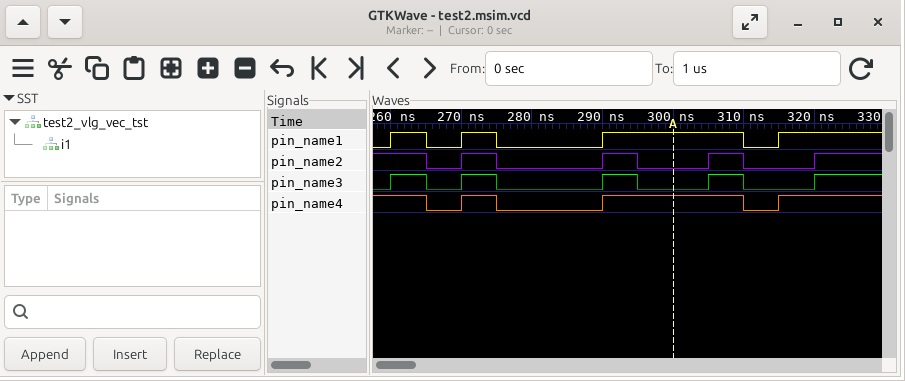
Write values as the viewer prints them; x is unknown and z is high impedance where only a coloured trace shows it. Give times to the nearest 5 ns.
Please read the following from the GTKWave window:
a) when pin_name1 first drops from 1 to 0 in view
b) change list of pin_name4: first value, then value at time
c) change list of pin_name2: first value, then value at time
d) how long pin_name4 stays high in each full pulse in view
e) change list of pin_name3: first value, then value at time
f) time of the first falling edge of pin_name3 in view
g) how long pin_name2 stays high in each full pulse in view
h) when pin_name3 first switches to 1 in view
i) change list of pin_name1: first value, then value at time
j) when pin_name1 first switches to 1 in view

265 ns
1, 0 at 265 ns, 1 at 270 ns, 0 at 275 ns, 1 at 290 ns, 0 at 310 ns, 1 at 315 ns
1, 0 at 265 ns, 1 at 270 ns, 0 at 275 ns, 1 at 290 ns, 0 at 295 ns, 1 at 305 ns, 0 at 310 ns, 1 at 320 ns
5 ns, 20 ns
0, 1 at 260 ns, 0 at 265 ns, 1 at 270 ns, 0 at 275 ns, 1 at 290 ns, 0 at 295 ns, 1 at 305 ns, 0 at 310 ns, 1 at 320 ns
265 ns
5 ns, 5 ns, 5 ns
260 ns
0, 1 at 260 ns, 0 at 265 ns, 1 at 270 ns, 0 at 275 ns, 1 at 290 ns, 0 at 310 ns, 1 at 315 ns
260 ns
